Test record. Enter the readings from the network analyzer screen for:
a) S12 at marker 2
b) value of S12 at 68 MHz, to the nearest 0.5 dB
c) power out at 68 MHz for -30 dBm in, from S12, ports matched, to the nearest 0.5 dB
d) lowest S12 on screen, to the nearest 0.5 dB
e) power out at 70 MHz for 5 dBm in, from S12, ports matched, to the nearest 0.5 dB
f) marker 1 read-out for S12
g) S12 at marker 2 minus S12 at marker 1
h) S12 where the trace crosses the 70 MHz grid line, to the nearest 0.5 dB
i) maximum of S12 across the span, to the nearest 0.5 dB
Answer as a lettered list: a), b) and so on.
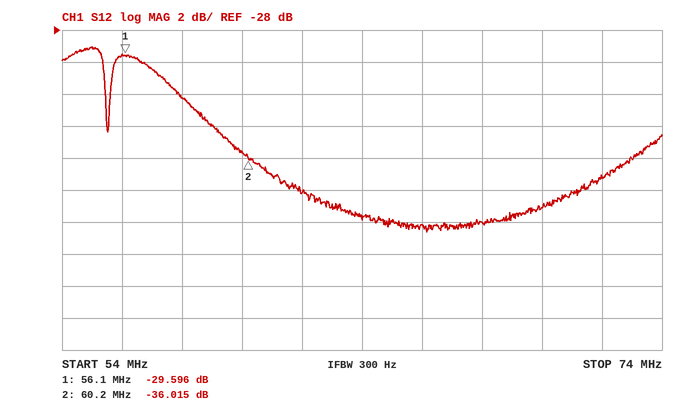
a) -36.015 dB
b) -40.0 dB
c) -70.0 dBm
d) -40.5 dB
e) -34.0 dBm
f) -29.596 dB
g) -6.419 dB
h) -39.0 dB
i) -29.0 dB
